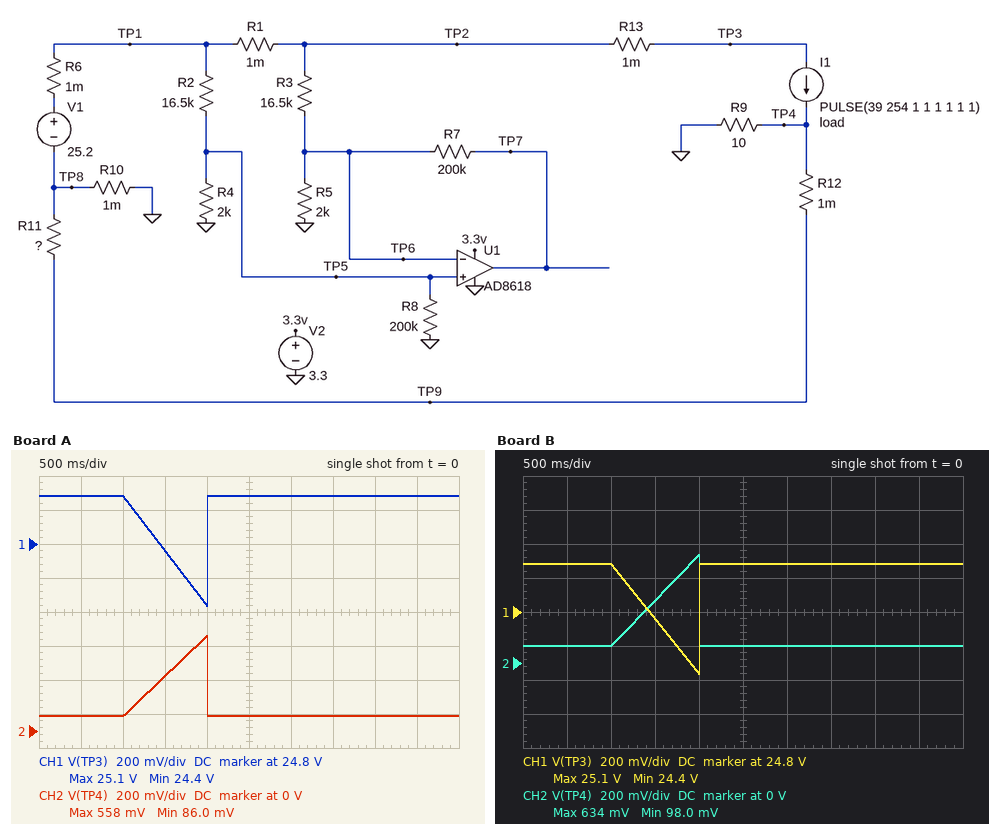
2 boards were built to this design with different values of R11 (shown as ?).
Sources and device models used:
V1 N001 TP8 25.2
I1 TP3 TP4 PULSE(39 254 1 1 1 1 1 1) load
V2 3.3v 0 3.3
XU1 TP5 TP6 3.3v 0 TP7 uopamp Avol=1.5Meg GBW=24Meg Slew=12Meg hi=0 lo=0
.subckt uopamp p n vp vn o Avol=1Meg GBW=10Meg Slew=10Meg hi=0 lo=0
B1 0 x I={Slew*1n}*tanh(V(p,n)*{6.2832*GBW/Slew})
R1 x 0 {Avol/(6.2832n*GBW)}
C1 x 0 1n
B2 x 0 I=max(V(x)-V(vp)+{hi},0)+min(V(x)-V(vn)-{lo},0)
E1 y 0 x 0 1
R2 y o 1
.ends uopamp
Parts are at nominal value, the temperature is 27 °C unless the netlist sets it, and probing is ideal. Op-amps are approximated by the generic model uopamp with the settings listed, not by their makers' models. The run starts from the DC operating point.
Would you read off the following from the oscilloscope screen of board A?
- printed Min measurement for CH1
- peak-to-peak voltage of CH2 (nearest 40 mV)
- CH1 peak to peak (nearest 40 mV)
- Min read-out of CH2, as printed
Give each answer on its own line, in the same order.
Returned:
24.4 V
480 mV
640 mV
86.0 mV
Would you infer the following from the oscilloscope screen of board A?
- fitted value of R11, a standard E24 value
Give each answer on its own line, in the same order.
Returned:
1.2 mΩ
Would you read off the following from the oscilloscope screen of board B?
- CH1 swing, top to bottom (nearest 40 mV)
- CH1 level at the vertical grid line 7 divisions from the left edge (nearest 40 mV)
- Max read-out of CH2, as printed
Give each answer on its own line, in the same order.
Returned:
640 mV
25.08 V
634 mV
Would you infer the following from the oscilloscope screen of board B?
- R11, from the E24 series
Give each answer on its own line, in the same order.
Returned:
1.5 mΩ
